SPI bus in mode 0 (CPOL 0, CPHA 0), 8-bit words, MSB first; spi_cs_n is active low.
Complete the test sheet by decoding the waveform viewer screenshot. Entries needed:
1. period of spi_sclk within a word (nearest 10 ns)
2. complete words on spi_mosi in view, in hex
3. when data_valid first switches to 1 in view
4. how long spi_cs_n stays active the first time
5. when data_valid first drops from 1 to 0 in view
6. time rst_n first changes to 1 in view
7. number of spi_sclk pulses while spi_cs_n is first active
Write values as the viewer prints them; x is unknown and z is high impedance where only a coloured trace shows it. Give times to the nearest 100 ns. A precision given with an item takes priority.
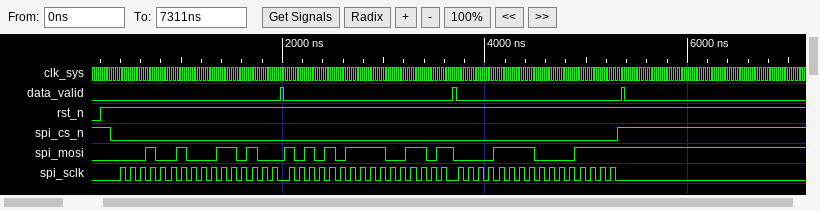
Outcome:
100 ns
12, 34, AB, CD, 0F, 0F
2000 ns
5000 ns
2000 ns
200 ns
48
